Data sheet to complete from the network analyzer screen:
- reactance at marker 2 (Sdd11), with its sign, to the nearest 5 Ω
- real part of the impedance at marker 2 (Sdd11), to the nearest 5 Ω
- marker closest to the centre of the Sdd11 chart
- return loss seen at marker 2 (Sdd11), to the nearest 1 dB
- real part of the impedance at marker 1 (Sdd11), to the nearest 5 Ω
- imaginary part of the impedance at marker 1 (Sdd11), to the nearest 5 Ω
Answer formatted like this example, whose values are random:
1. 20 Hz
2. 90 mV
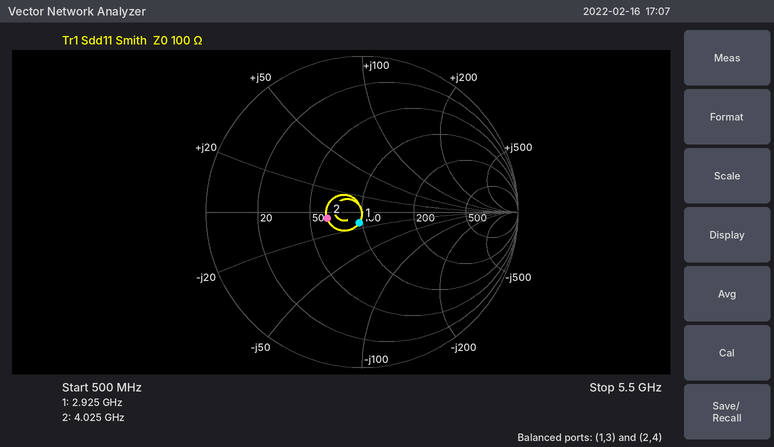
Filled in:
1. -5 Ω
2. 65 Ω
3. marker 1
4. 13 dB
5. 95 Ω
6. -15 Ω
